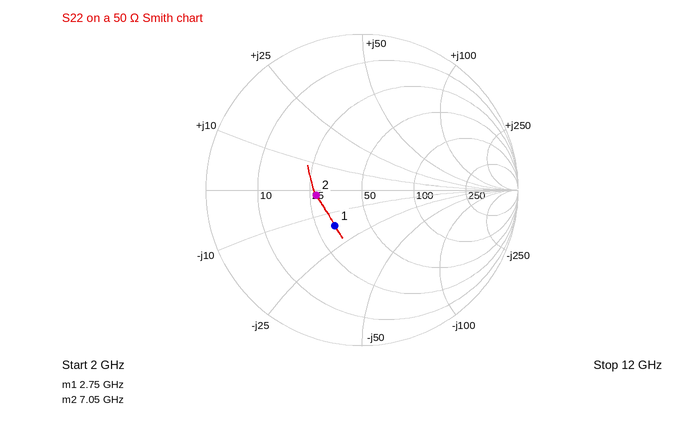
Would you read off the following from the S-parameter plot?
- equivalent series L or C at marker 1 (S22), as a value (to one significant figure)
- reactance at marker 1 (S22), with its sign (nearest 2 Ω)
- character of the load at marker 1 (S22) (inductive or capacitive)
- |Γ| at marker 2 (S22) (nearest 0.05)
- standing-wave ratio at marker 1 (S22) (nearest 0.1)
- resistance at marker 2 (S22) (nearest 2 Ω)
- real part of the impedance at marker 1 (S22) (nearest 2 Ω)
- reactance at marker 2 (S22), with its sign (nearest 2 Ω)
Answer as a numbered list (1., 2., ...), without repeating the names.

1. 4 pF
2. -16 Ω
3. capacitive
4. 0.30
5. 1.8
6. 28 Ω
7. 32 Ω
8. -2 Ω
